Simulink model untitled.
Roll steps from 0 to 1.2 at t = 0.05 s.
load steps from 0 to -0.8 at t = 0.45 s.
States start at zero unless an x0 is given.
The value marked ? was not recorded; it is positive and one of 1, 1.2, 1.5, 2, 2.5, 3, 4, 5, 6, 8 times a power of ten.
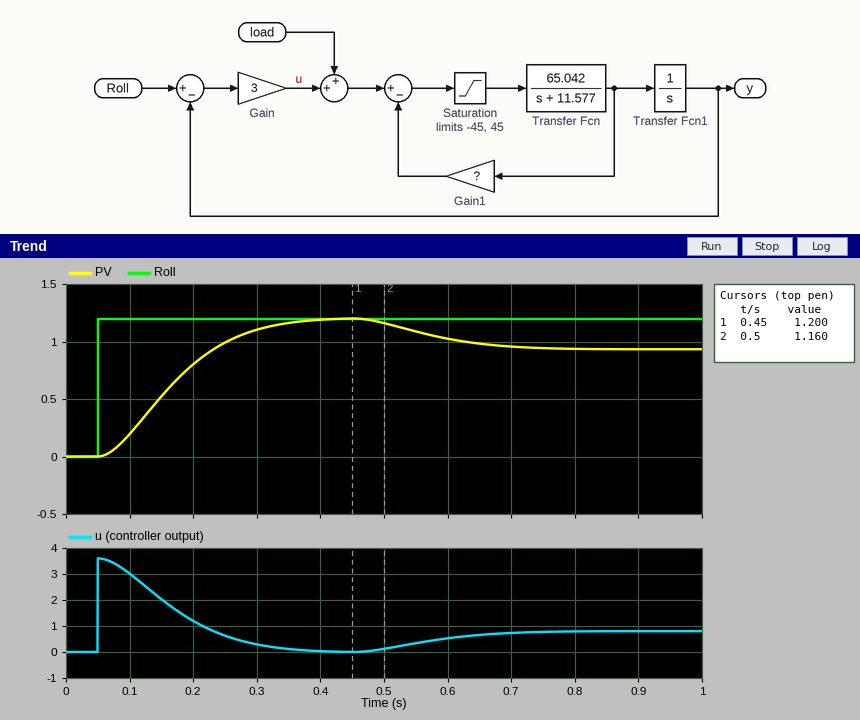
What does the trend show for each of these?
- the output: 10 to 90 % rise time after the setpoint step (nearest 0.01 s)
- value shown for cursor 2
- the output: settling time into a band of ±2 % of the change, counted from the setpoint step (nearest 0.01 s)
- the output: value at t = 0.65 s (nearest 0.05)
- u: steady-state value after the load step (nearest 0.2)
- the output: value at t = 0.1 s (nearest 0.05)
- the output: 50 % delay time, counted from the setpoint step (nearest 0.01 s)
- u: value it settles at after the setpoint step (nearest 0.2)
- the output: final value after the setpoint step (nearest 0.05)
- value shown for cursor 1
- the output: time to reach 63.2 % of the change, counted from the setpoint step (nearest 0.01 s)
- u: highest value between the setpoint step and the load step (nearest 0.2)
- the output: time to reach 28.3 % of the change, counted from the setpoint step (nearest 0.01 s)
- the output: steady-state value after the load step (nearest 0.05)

0.20 s
1.160
0.32 s
1.00
0.8
0.20
0.11 s
0.0
1.20
1.200
0.14 s
3.6
0.07 s
0.95
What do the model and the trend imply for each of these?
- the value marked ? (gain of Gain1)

0.2
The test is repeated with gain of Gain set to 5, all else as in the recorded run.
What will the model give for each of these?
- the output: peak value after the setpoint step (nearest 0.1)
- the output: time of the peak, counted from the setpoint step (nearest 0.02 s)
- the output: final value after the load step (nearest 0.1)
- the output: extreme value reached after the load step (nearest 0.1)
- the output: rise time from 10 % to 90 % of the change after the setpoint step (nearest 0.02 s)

1.3
0.24 s
1.0
1.0
0.12 s
